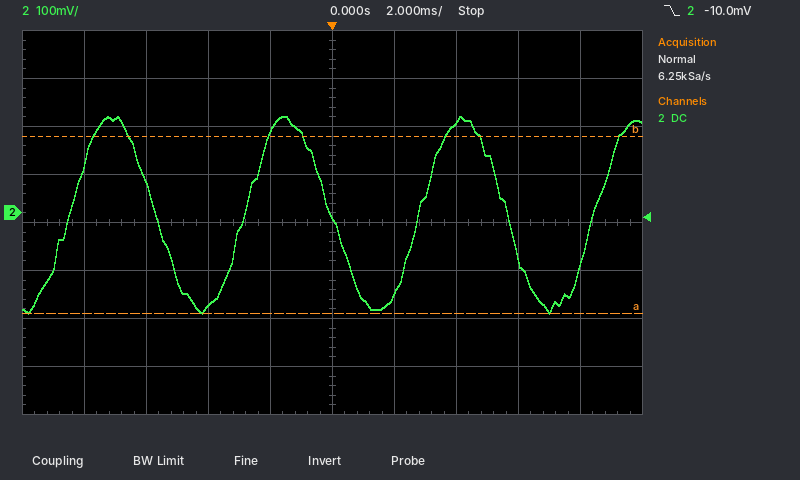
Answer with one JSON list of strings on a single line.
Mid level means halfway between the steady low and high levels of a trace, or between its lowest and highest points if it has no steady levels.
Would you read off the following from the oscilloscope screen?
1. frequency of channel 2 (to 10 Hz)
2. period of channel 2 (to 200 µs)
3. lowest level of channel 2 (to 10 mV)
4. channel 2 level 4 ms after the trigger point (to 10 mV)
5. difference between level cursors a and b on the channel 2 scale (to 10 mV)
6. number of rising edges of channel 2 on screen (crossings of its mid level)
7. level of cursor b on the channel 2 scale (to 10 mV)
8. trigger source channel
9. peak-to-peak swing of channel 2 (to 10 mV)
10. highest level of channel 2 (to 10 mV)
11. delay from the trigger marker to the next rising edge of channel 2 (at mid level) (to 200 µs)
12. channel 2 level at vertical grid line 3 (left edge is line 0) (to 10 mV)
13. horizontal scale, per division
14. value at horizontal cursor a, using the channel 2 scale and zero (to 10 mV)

["180 Hz", "5.6 ms", "-210 mV", "190 mV", "370 mV", "4", "160 mV", "channel 2", "410 mV", "200 mV", "2.8 ms", "-190 mV", "2 ms", "-210 mV"]
